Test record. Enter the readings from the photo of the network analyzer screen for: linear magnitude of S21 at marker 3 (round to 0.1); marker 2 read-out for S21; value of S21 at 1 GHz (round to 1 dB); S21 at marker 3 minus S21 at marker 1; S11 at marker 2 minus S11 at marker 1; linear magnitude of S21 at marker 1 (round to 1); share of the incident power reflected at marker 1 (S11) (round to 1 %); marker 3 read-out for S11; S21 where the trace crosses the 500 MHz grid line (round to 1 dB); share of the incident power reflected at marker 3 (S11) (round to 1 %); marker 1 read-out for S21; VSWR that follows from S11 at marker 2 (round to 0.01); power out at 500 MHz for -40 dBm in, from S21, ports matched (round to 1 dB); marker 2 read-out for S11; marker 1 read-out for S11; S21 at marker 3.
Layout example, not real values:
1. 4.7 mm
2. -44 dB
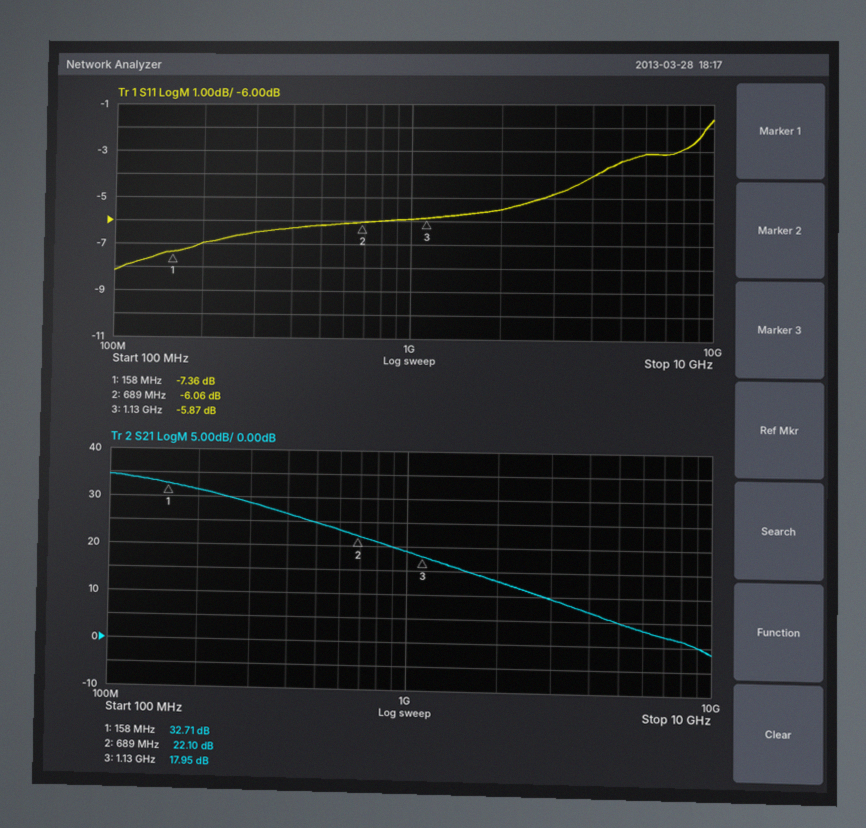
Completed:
1. 7.9
2. 22.10 dB
3. 19 dB
4. -14.76 dB
5. 1.30 dB
6. 43
7. 18 %
8. -5.87 dB
9. 25 dB
10. 26 %
11. 32.71 dB
12. 2.98
13. -15 dBm
14. -6.06 dB
15. -7.36 dB
16. 17.95 dB
